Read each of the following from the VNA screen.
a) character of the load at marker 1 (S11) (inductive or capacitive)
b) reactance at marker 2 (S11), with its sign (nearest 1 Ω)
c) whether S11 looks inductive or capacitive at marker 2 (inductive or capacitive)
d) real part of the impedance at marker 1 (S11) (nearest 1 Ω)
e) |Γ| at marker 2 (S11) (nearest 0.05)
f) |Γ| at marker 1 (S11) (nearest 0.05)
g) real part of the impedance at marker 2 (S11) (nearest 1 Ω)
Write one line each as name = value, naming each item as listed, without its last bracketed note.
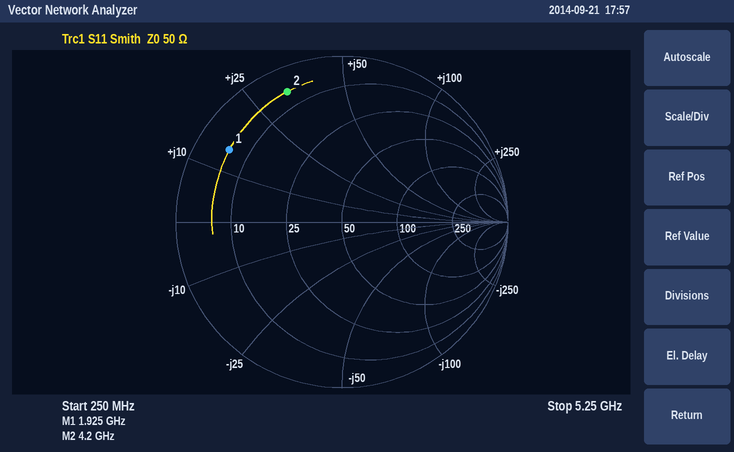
character of the load at marker 1 (S11) = inductive
reactance at marker 2 (S11), with its sign = +33 Ω
whether S11 looks inductive or capacitive at marker 2 = inductive
real part of the impedance at marker 1 (S11) = 6 Ω
|Γ| at marker 2 (S11) = 0.85
|Γ| at marker 1 (S11) = 0.80
real part of the impedance at marker 2 (S11) = 6 Ω
